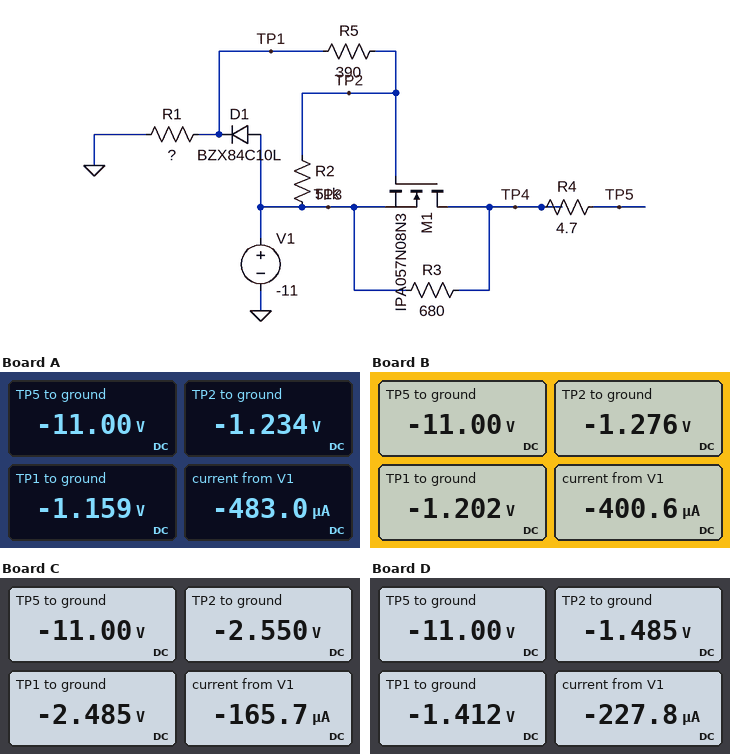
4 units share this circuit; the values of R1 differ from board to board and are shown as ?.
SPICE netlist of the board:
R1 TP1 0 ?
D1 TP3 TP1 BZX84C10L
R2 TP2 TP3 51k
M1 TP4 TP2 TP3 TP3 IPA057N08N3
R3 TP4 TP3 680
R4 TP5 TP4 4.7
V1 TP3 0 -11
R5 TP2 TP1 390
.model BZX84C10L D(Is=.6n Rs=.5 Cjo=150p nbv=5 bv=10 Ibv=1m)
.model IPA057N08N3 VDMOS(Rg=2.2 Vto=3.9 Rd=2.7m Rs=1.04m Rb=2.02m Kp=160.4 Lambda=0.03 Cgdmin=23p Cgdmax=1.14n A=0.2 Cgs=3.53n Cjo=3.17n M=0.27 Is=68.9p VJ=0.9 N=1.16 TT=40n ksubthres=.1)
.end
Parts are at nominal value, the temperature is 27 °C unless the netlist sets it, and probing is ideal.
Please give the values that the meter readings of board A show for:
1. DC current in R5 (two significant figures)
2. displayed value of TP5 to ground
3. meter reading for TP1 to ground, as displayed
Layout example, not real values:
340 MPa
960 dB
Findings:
190 µA
-11.00 V
-1.159 V
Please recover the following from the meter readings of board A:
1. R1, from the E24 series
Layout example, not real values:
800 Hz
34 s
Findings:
2.4 kΩ
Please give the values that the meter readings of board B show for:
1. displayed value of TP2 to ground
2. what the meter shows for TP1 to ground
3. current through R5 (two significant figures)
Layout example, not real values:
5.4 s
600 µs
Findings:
-1.276 V
-1.202 V
190 µA
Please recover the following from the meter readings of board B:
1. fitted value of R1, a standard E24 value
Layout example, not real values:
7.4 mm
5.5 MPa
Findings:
3 kΩ
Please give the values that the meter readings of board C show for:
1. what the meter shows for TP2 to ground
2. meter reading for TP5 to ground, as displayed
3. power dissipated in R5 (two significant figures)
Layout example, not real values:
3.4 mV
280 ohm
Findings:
-2.550 V
-11.00 V
11 µW
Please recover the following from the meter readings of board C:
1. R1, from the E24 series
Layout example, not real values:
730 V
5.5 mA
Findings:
15 kΩ
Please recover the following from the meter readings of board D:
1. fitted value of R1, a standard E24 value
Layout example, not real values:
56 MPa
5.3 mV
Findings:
6.2 kΩ
